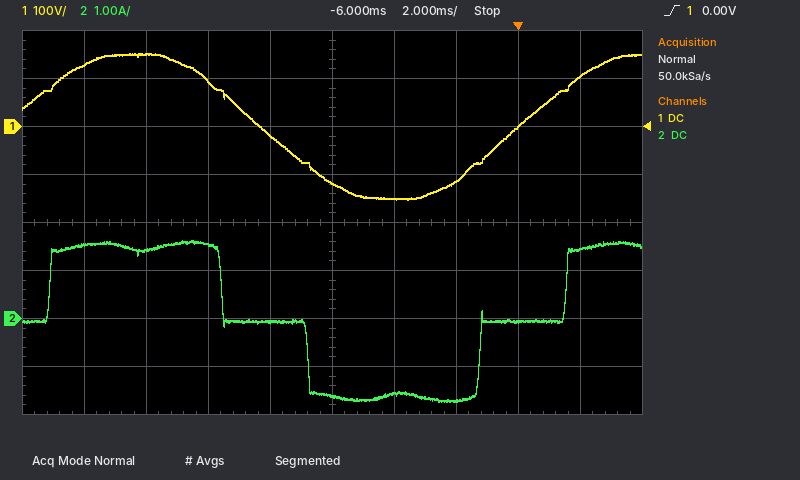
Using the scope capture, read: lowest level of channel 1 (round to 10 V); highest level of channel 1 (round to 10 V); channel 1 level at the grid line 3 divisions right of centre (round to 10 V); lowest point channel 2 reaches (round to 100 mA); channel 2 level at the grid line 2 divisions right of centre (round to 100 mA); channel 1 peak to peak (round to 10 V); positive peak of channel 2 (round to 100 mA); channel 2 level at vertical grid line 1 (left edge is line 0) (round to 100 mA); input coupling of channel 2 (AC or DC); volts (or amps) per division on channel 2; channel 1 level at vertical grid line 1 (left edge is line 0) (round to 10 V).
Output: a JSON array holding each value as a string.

["-150 V", "150 V", "0 V", "-1.7 A", "-1.7 A", "300 V", "1.6 A", "1.5 A", "DC", "1 A", "130 V"]
